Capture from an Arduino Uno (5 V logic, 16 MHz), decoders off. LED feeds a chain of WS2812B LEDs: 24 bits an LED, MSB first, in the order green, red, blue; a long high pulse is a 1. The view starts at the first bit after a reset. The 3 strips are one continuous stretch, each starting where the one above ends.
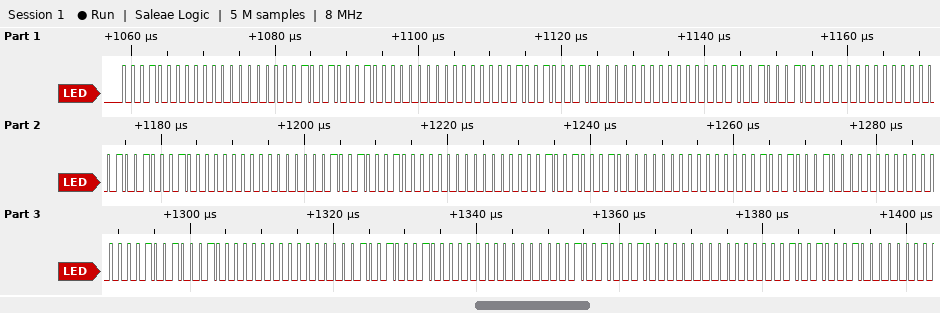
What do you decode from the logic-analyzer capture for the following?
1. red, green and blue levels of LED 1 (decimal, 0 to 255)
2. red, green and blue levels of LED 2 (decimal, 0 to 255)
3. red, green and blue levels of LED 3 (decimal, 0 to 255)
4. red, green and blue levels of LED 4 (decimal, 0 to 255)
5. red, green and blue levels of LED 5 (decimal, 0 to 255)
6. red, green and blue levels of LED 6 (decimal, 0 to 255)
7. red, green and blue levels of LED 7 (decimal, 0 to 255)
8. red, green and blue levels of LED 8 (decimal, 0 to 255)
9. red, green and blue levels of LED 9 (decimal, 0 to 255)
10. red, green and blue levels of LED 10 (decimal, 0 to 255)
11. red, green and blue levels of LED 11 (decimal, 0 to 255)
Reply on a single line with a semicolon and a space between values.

0, 16, 9; 0, 16, 9; 0, 16, 9; 0, 16, 9; 0, 16, 9; 0, 16, 9; 0, 16, 9; 0, 16, 9; 0, 16, 9; 0, 16, 9; 0, 16, 9
